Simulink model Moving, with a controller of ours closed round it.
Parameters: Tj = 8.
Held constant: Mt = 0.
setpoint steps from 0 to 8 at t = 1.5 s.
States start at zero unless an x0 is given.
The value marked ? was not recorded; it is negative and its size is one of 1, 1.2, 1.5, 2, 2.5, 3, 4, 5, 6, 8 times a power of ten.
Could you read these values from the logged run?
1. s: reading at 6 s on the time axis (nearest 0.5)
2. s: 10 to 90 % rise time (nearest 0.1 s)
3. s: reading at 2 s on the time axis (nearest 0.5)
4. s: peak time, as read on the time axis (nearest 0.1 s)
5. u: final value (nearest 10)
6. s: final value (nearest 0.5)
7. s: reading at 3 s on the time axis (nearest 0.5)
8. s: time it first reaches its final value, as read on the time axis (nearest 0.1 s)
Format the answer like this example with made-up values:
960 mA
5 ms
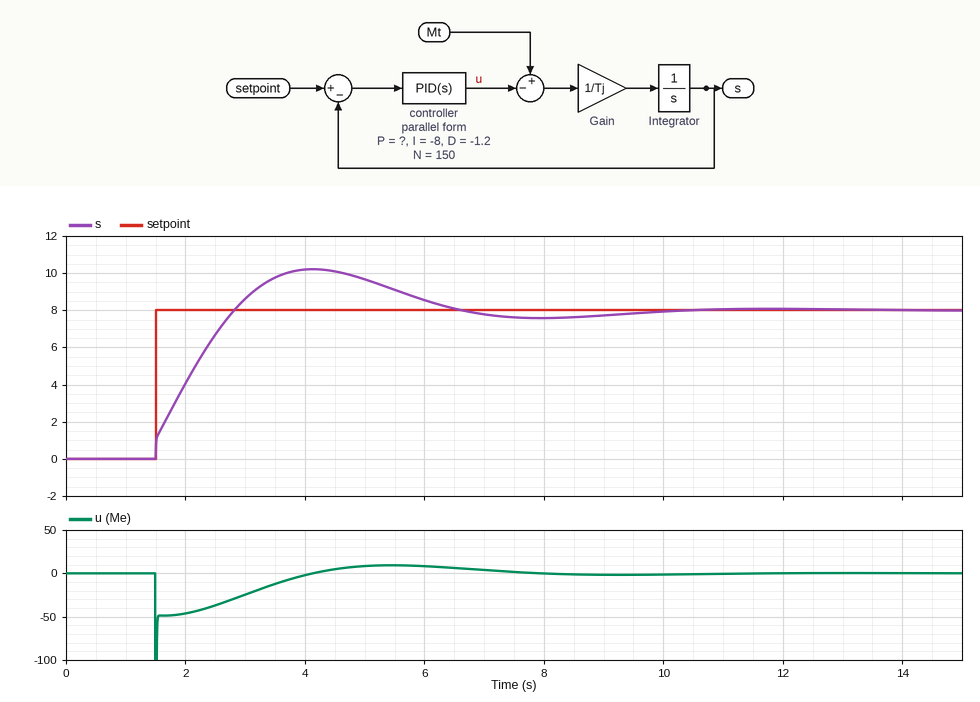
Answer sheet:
8.5
1.1 s
4.0
4.1 s
0
8.0
8.5
2.8 s
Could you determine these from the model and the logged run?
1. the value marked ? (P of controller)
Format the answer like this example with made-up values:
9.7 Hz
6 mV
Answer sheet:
-8
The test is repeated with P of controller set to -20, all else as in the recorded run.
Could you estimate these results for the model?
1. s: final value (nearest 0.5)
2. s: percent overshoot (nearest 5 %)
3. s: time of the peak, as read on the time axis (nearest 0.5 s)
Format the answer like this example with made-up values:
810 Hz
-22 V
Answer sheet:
8.0
10 %
3.5 s
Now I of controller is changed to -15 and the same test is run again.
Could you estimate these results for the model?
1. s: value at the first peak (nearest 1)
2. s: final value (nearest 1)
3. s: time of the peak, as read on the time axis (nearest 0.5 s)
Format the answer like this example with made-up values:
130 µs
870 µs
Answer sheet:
11
8
3.5 s
